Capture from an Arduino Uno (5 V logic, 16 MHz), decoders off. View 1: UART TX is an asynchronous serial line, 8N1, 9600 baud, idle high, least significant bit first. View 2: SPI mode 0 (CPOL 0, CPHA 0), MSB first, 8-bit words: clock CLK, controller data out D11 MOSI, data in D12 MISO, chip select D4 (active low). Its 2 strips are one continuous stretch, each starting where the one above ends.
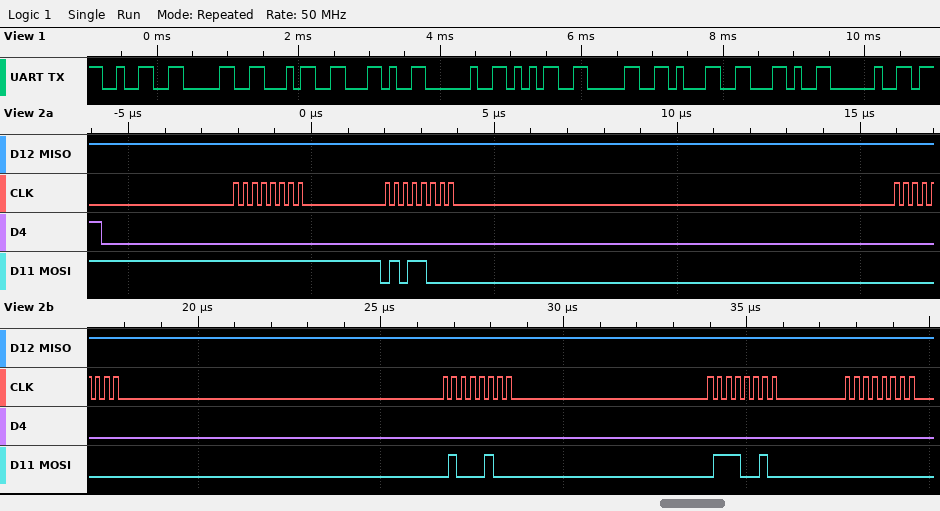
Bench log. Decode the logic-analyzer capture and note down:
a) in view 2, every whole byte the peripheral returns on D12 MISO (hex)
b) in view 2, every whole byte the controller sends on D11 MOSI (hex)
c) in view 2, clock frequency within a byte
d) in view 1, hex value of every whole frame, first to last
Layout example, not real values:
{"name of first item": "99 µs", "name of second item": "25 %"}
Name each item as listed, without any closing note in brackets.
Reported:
{"in view 2, every whole byte the peripheral returns on D12 MISO": "FF FF FF FF FF FF", "in view 2, every whole byte the controller sends on D11 MOSI": "FF 58 00 44 72 00", "in view 2, clock frequency within a byte": "4 MHz", "in view 1, hex value of every whole frame, first to last": "32 30 34 2C 20 35 30 31 2C 20"}
